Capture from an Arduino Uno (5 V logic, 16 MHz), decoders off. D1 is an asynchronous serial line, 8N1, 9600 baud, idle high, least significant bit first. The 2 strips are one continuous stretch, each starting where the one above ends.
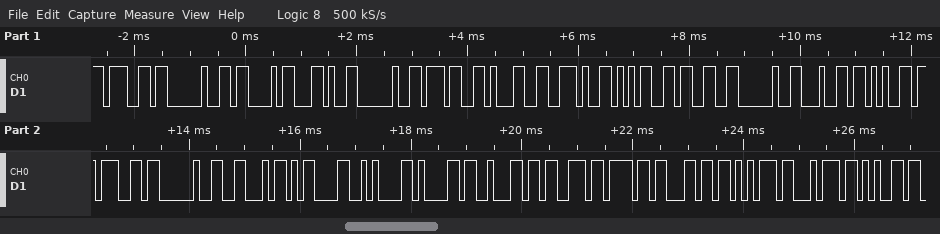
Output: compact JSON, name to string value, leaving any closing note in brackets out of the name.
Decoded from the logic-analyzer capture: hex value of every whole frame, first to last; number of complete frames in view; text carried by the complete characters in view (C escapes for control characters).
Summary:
{"hex value of every whole frame, first to last": "67 20 43 2C 20 37 31 2E 35 33 20 64 65 67 20 46 0D 0A 61 62 73 6F 6C 75 74 65", "number of complete frames in view": "26", "text carried by the complete characters in view": "\"g C, 71.53 deg F\\r\\nabsolute\""}
